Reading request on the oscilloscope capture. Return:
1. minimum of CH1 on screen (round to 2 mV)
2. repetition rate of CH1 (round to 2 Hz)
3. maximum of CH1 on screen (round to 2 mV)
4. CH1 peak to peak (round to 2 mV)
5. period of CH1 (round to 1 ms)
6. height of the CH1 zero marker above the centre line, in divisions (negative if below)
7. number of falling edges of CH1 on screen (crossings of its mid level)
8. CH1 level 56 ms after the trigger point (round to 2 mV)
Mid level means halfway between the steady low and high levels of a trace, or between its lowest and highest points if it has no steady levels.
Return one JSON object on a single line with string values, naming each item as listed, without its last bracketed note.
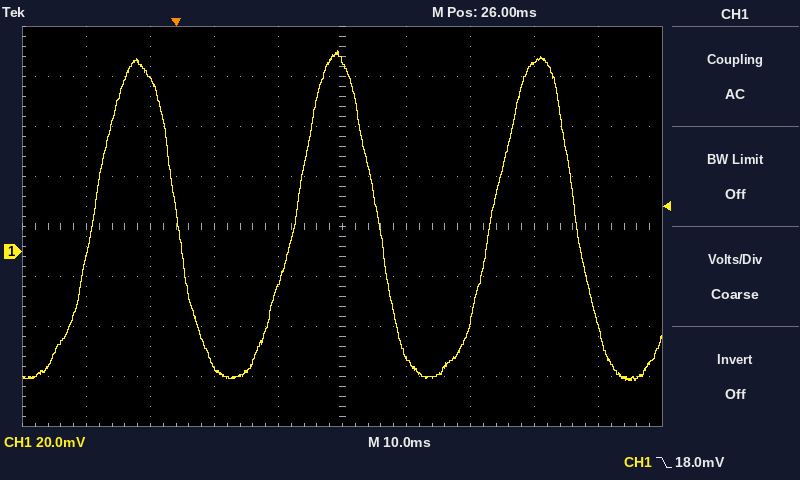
{"minimum of CH1 on screen": "-52 mV", "repetition rate of CH1": "32 Hz", "maximum of CH1 on screen": "80 mV", "CH1 peak to peak": "132 mV", "period of CH1": "31 ms", "height of the CH1 zero marker above the centre line, in divisions": "-0.5 div", "number of falling edges of CH1 on screen": "3", "CH1 level 56 ms after the trigger point": "76 mV"}
